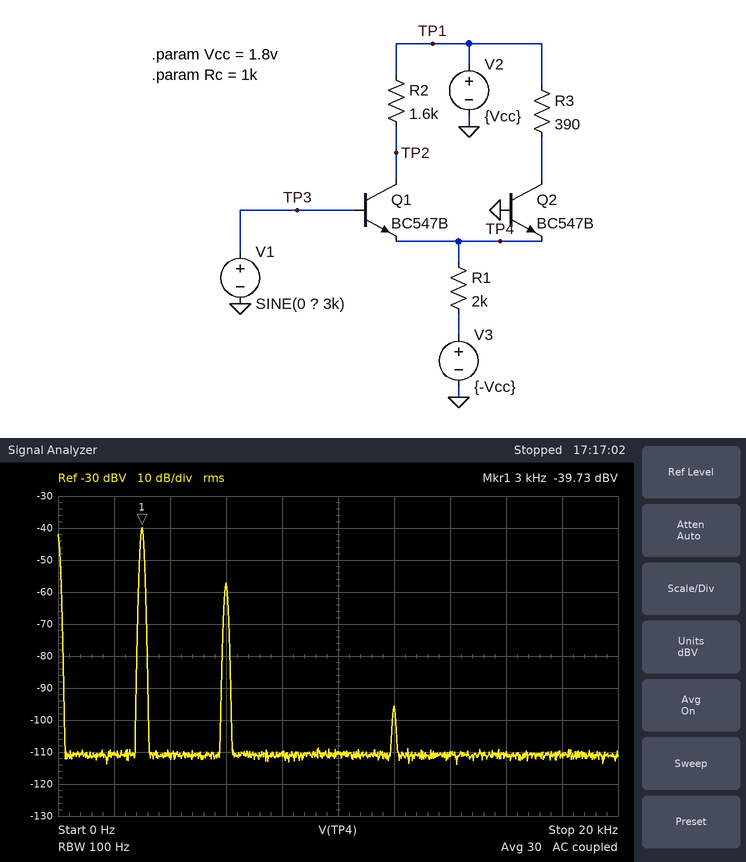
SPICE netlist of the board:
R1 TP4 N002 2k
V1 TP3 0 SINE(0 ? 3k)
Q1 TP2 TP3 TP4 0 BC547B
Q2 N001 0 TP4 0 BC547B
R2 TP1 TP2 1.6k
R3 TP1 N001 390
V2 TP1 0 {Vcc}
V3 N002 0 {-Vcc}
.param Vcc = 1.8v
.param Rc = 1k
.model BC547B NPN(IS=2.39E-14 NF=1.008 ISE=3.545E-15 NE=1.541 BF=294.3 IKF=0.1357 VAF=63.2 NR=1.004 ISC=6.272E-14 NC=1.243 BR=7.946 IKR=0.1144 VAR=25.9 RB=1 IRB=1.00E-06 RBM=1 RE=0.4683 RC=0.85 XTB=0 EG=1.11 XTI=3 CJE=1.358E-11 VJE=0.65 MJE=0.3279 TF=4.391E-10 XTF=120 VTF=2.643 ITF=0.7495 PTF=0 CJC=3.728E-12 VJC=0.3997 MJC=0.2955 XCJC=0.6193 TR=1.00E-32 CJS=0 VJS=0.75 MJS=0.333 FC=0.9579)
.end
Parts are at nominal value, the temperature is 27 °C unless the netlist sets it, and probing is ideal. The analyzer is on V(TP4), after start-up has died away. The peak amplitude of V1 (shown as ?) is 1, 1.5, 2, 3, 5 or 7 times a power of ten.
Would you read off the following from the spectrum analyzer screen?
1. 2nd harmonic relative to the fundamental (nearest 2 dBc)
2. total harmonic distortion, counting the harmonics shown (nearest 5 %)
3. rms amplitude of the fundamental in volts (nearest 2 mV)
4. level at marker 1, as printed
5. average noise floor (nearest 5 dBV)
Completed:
-18 dBc
15 %
10 mV
-39.73 dBV
-110 dBV
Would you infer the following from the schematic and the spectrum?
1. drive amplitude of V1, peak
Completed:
30 mV
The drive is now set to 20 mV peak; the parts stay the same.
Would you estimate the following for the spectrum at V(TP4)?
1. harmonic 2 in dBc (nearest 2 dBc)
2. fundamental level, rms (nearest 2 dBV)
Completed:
-20 dBc
-44 dBV
